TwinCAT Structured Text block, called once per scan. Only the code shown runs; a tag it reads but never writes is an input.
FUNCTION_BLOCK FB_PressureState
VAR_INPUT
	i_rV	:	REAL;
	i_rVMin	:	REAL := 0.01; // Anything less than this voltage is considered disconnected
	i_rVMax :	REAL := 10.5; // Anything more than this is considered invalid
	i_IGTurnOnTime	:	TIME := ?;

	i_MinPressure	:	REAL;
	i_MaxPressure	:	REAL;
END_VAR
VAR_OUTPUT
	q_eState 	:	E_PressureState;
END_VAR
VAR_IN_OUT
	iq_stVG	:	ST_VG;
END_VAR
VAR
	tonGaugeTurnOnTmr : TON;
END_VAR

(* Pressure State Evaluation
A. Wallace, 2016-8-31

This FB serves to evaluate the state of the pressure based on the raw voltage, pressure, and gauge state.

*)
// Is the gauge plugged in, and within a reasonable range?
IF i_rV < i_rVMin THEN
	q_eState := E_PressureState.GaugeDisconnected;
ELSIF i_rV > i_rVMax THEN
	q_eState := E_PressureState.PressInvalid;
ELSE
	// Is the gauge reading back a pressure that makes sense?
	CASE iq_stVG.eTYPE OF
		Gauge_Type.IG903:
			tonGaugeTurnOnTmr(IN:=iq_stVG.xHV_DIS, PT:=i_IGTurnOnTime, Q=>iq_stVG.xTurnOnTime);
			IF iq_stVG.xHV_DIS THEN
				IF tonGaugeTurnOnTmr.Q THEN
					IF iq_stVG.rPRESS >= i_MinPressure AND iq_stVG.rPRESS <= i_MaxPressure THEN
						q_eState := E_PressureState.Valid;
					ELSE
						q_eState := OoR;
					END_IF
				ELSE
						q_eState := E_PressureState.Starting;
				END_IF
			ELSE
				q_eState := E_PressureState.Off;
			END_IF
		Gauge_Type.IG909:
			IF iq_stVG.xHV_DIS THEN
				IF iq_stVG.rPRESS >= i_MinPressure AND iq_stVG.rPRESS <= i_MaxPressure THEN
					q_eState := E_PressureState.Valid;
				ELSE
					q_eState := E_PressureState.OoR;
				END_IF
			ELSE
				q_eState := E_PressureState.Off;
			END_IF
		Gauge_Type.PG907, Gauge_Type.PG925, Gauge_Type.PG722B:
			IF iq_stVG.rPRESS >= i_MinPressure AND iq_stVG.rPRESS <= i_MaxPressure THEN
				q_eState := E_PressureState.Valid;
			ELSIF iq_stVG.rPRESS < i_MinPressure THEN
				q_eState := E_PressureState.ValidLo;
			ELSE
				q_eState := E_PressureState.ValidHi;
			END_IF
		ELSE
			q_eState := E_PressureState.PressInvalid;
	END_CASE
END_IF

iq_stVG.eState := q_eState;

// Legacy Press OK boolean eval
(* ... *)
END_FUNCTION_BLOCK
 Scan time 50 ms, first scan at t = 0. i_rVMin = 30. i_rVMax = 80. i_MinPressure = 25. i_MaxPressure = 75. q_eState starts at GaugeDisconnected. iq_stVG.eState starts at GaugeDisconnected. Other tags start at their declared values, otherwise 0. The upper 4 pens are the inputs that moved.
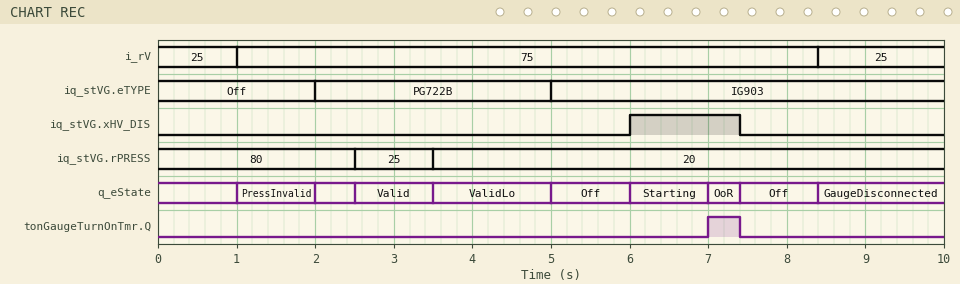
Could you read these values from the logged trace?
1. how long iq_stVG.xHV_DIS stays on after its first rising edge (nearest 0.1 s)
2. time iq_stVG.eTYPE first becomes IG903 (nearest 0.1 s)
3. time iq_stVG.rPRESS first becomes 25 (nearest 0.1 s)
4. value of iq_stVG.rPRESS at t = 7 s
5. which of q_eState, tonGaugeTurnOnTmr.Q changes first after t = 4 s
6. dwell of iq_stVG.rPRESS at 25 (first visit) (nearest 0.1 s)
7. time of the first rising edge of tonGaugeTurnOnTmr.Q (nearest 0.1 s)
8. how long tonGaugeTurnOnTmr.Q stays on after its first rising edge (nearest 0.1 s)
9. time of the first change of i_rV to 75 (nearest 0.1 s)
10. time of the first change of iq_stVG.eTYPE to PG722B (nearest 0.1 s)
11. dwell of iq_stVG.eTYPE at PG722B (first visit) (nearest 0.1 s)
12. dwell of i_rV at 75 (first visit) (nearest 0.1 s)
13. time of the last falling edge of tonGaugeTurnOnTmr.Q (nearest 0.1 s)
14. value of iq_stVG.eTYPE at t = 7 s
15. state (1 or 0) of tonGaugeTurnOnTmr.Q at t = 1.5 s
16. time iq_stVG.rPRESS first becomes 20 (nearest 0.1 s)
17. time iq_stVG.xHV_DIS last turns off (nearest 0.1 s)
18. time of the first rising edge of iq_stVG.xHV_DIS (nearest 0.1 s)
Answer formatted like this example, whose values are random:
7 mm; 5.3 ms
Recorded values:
1.4 s; 5.0 s; 2.5 s; 20; q_eState; 1.0 s; 7.0 s; 0.4 s; 1.0 s; 2.0 s; 3.0 s; 7.4 s; 7.4 s; IG903; 0; 3.5 s; 7.4 s; 6.0 s
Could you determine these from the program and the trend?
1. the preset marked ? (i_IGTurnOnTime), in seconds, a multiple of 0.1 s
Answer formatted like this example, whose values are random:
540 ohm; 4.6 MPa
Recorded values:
1.0 s
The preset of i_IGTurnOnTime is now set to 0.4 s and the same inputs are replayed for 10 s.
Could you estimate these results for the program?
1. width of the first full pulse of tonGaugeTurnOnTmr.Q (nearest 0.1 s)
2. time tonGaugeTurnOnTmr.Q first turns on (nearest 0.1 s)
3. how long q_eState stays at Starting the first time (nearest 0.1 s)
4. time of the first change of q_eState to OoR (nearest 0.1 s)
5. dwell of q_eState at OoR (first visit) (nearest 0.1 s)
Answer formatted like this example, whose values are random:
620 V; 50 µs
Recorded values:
1.0 s; 6.4 s; 0.4 s; 6.4 s; 1.0 s
